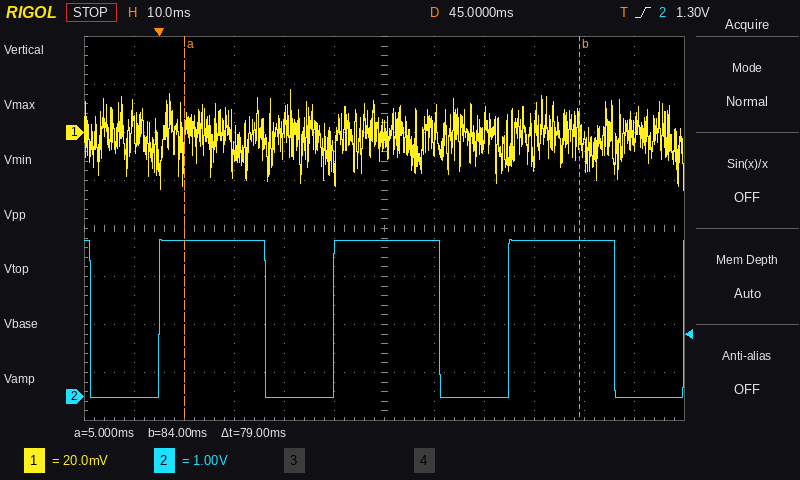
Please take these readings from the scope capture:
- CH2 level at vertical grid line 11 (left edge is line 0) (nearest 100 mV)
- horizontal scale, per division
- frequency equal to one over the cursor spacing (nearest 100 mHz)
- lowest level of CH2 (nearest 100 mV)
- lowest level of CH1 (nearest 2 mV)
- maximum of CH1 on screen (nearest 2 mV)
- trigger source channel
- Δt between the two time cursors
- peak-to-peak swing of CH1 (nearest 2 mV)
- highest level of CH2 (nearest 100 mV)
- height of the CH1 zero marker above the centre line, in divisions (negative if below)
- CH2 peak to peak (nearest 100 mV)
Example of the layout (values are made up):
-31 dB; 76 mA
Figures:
0.0 V; 10 ms; 12.7 Hz; 0.0 V; -24 mV; 18 mV; CH2; 79 ms; 42 mV; 3.3 V; +2.0 div; 3.3 V
